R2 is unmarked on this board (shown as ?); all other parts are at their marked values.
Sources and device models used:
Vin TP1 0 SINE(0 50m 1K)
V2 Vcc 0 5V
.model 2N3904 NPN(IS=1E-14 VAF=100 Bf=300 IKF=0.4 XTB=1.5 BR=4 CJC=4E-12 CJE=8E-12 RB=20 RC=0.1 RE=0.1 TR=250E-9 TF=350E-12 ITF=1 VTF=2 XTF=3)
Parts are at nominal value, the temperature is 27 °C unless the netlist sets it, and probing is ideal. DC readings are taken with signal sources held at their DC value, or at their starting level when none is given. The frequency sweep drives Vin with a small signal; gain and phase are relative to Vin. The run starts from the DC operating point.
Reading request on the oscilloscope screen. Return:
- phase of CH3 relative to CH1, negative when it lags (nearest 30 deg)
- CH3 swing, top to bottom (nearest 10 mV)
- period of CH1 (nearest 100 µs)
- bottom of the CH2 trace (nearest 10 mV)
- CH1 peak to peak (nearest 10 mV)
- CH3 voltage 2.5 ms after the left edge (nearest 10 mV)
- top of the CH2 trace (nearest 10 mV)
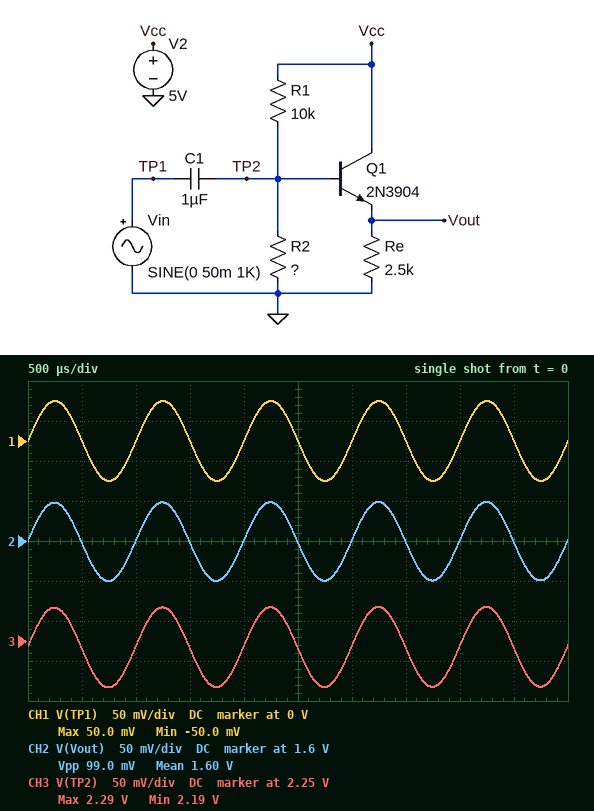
0 deg
100 mV
1.0 ms
1.55 V
100 mV
2.24 V
1.65 V
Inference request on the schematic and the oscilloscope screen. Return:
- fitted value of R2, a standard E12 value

8.2 kΩ
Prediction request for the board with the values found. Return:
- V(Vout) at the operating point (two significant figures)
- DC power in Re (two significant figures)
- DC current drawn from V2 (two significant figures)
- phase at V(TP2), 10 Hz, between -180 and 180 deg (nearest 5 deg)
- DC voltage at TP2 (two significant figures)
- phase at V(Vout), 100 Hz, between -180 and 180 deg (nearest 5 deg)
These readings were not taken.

1.6 V
1.0 mW
910 µA
75 deg
2.2 V
20 deg
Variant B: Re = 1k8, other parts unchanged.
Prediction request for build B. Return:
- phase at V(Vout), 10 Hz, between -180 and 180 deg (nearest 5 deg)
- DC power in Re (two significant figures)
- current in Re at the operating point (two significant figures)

75 deg
1.4 mW
880 µA
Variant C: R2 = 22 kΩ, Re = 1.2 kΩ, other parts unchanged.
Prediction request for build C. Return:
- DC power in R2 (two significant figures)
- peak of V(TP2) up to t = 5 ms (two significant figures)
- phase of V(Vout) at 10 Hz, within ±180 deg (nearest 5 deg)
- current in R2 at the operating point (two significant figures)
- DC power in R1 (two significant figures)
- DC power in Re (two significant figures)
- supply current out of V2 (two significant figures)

520 µW
3.4 V
65 deg
150 µA
260 µW
6.1 mW
2.4 mA
